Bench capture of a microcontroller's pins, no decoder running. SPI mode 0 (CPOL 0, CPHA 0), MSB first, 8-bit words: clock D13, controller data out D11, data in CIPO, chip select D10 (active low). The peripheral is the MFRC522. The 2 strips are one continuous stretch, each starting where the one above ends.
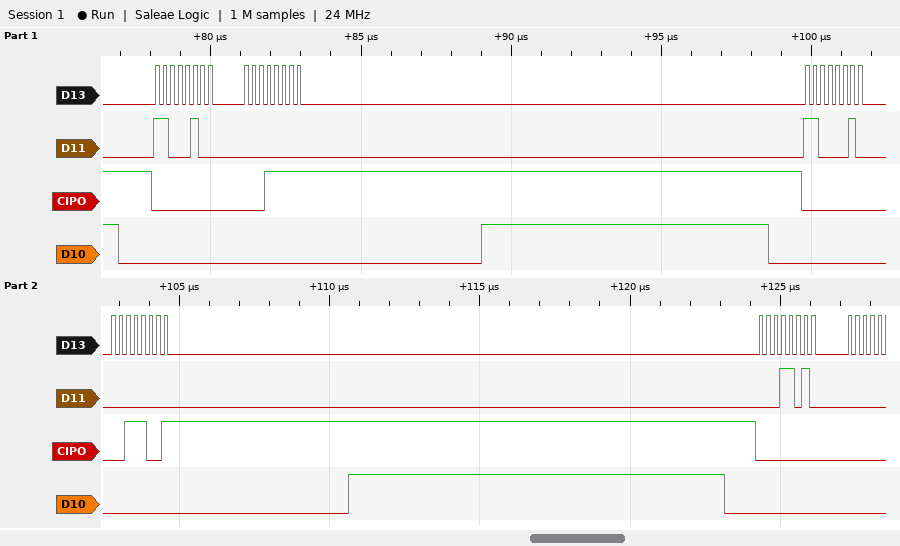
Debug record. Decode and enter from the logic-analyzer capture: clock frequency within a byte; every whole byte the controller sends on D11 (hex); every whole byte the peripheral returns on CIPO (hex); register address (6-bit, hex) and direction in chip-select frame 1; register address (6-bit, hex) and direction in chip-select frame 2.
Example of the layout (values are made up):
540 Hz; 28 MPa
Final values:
4 MHz; C4 00 C2 00 1A; 00 1F 00 39 00; 0x22 read; 0x21 read
